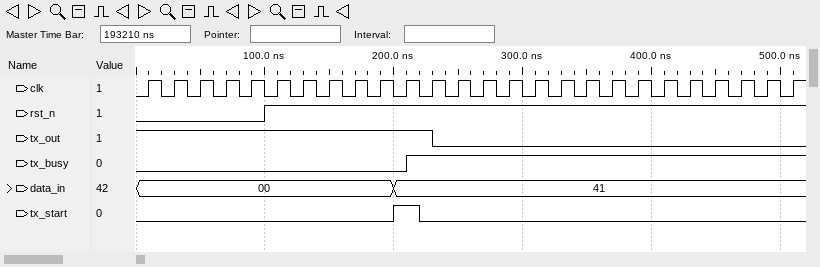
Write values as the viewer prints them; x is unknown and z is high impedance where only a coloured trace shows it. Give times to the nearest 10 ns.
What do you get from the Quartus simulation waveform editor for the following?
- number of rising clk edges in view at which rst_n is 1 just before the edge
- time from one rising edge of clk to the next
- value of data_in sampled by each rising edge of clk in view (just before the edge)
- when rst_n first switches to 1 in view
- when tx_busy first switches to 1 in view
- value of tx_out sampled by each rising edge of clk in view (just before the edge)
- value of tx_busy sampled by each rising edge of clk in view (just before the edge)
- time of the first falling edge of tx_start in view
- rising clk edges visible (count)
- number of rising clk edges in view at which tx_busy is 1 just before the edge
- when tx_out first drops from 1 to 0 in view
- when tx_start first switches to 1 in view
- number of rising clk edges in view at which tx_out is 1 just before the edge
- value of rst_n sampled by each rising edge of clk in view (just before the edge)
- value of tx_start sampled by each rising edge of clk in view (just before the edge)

21
20 ns
00, 00, 00, 00, 00, 00, 00, 00, 00, 00, 41, 41, 41, 41, 41, 41, 41, 41, 41, 41, 41, 41, 41, 41, 41, 41
100 ns
210 ns
1 1 1 1 1 1 1 1 1 1 1 1 0 0 0 0 0 0 0 0 0 0 0 0 0 0
0 0 0 0 0 0 0 0 0 0 0 1 1 1 1 1 1 1 1 1 1 1 1 1 1 1
220 ns
26
15
230 ns
200 ns
12
0 0 0 0 0 1 1 1 1 1 1 1 1 1 1 1 1 1 1 1 1 1 1 1 1 1
0 0 0 0 0 0 0 0 0 0 1 0 0 0 0 0 0 0 0 0 0 0 0 0 0 0
